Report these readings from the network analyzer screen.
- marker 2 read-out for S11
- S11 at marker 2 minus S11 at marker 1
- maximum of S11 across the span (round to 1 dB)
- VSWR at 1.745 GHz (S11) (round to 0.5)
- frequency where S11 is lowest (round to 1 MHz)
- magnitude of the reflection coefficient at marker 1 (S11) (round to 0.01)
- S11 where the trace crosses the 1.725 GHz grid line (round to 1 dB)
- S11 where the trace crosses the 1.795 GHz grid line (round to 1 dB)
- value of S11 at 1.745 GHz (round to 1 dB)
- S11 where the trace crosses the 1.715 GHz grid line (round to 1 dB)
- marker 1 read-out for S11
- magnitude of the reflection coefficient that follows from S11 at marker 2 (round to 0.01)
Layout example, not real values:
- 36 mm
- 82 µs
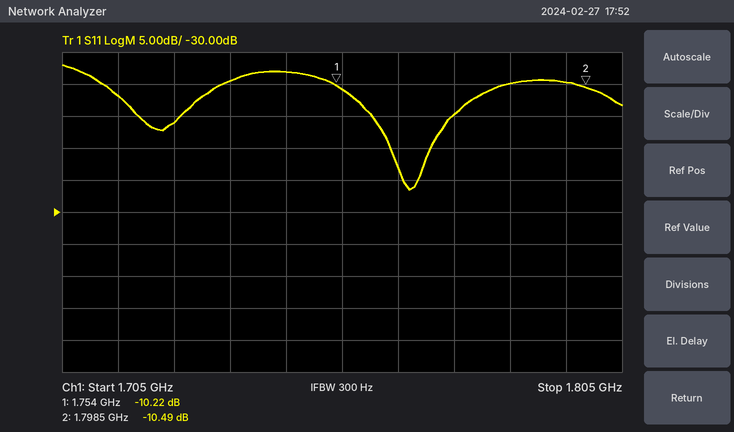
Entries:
- -10.49 dB
- -0.27 dB
- -7 dB
- 2.5
- 1.767 GHz
- 0.31
- -16 dB
- -10 dB
- -8 dB
- -12 dB
- -10.22 dB
- 0.30
